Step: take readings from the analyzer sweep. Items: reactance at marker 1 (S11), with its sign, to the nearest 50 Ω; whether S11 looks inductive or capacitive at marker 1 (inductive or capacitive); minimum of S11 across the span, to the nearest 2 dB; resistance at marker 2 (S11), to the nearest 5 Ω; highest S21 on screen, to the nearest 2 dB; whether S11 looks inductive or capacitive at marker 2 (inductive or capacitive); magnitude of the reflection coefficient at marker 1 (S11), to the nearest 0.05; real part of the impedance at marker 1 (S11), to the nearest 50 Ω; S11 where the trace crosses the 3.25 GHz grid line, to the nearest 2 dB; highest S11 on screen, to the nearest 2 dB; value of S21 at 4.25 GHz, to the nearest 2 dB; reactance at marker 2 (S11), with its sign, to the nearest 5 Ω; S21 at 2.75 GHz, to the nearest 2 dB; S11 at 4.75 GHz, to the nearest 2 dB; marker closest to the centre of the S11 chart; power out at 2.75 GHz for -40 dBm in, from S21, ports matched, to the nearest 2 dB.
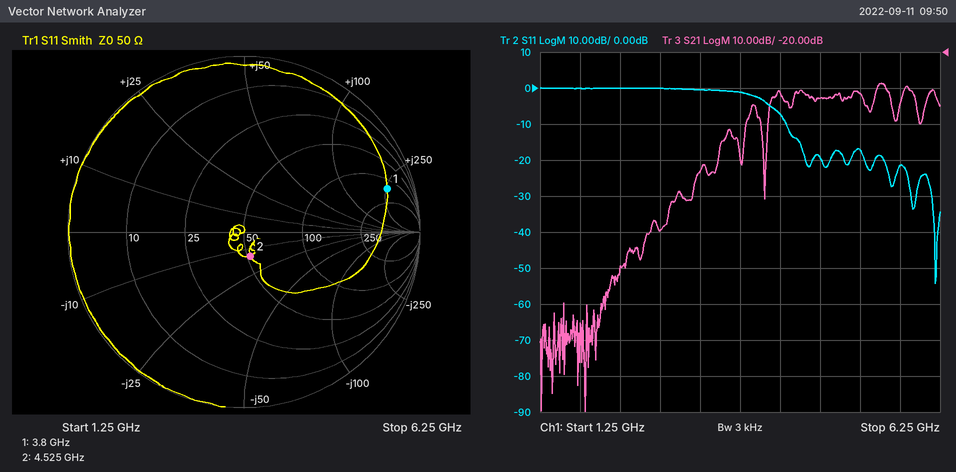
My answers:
+250 Ω
inductive
-54 dB
50 Ω
-28 dB
capacitive
0.85
150 Ω
0 dB
0 dB
-32 dB
-15 Ω
-70 dB
-20 dB
marker 2
-110 dBm
